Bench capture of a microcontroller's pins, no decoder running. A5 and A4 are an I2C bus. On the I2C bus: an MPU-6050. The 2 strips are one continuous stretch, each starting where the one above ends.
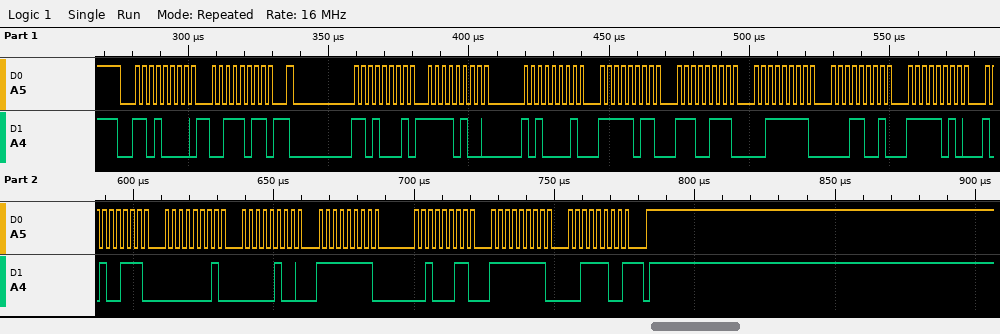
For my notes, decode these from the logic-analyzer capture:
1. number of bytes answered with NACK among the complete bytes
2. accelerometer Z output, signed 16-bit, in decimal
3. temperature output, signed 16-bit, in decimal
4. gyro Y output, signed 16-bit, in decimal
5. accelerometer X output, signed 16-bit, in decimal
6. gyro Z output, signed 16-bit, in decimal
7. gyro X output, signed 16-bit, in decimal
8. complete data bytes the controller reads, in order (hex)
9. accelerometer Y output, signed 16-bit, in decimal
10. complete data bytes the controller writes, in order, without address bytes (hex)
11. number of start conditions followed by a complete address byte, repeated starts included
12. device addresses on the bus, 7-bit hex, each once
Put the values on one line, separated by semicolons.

1; 16153; -1369; -221; -2911; -196; 260; F4 A1 FB E7 3F 19 FA A7 01 04 FF 23 FF 3C; -1049; 3B; 2; 0x68
